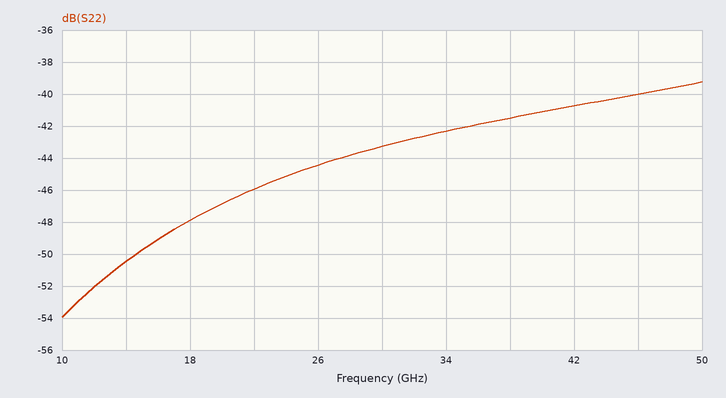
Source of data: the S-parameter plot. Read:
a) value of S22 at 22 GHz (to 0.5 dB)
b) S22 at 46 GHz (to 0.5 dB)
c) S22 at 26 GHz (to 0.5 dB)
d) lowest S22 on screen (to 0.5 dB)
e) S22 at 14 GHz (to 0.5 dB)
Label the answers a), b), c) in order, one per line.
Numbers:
a) -46.0 dB
b) -40.0 dB
c) -44.5 dB
d) -54.0 dB
e) -50.5 dB
